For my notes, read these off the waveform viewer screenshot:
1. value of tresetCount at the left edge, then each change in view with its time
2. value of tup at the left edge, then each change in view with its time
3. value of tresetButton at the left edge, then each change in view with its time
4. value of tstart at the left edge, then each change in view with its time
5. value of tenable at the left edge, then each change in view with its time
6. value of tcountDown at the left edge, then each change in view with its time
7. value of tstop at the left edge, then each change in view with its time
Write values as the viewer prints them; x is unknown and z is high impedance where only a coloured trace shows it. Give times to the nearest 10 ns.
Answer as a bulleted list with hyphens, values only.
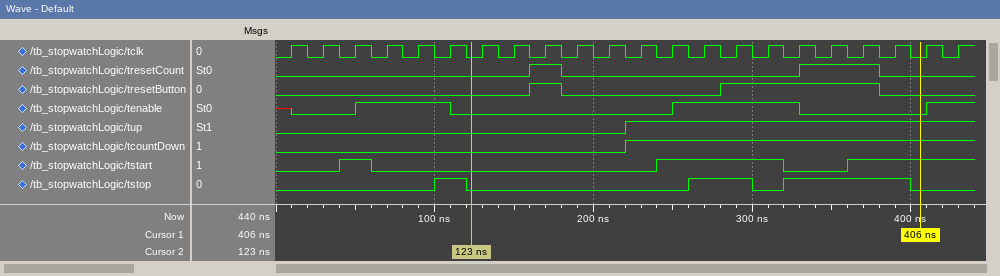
- 0, 1 at 160 ns, 0 at 180 ns, 1 at 330 ns, 0 at 380 ns
- 0, 1 at 220 ns
- 0, 1 at 160 ns, 0 at 180 ns, 1 at 280 ns, 0 at 380 ns
- 0, 1 at 40 ns, 0 at 60 ns, 1 at 240 ns, 0 at 320 ns, 1 at 360 ns
- x, 0 at 10 ns, 1 at 50 ns, 0 at 110 ns, 1 at 250 ns, 0 at 330 ns, 1 at 410 ns
- 0, 1 at 220 ns
- 0, 1 at 100 ns, 0 at 120 ns, 1 at 260 ns, 0 at 300 ns, 1 at 320 ns, 0 at 400 ns
